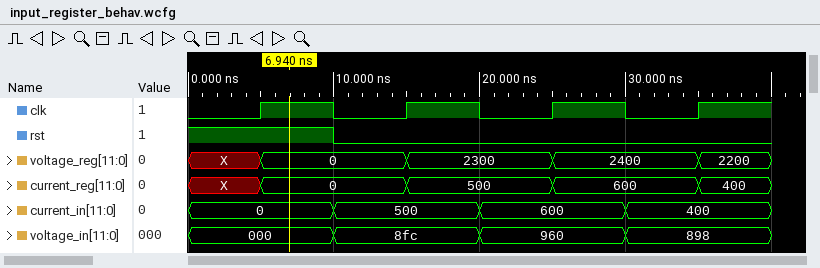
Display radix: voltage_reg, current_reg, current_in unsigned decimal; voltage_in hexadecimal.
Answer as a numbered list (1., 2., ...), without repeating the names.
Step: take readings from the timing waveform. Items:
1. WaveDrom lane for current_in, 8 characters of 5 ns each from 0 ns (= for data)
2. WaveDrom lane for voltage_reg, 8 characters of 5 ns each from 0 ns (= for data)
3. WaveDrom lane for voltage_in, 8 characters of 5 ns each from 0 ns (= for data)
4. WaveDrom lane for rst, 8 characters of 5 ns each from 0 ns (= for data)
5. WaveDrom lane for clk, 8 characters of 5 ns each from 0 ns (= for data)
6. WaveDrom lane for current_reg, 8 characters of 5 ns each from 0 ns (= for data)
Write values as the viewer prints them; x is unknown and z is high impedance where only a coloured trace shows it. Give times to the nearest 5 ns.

1. {name: 'current_in', wave: '=.=.=.=.', data: '0 500 600 400'}
2. {name: 'voltage_reg', wave: 'x=.=.=.=', data: '0 2300 2400 2200'}
3. {name: 'voltage_in', wave: '=.=.=.=.', data: '000 8fc 960 898'}
4. {name: 'rst', wave: '1.0.....'}
5. {name: 'clk', wave: '01010101'}
6. {name: 'current_reg', wave: 'x=.=.=.=', data: '0 500 600 400'}
